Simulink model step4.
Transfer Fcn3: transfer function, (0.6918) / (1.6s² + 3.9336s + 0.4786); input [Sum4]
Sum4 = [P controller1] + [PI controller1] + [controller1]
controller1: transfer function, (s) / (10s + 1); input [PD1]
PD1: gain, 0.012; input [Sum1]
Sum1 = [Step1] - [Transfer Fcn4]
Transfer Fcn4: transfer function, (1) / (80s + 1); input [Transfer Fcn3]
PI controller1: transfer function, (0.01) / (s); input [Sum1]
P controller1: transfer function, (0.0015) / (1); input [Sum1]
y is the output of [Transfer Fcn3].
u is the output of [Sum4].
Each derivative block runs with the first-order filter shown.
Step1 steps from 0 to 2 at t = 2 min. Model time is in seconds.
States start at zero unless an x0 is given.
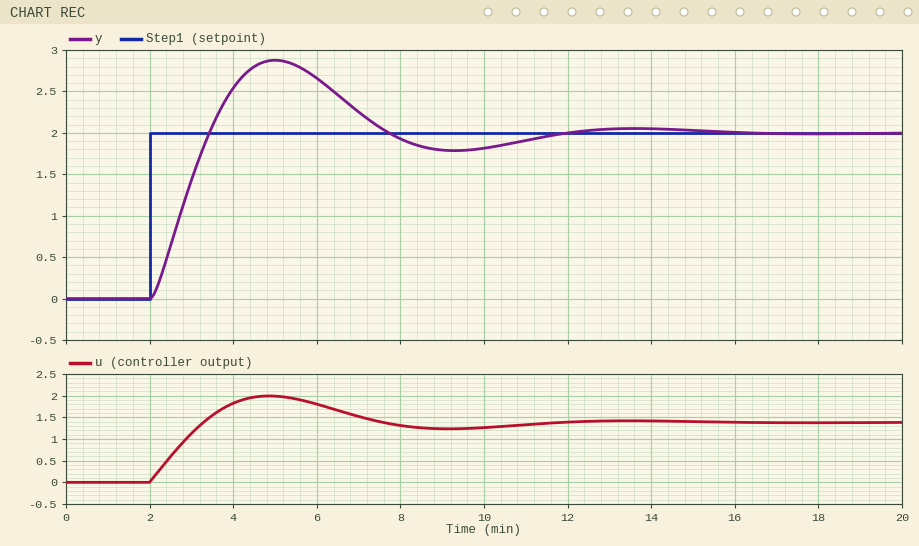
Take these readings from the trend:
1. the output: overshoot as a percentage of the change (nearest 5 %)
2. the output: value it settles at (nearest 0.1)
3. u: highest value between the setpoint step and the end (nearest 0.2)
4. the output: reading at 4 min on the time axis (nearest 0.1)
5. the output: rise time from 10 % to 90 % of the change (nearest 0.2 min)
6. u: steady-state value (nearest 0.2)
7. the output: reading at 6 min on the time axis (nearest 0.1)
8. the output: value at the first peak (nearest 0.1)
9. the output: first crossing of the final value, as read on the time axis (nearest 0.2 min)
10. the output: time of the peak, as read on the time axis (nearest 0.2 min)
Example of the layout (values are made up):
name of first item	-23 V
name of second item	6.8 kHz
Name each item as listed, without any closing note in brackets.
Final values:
the output: overshoot as a percentage of the change	45 %
the output: value it settles at	2.0
u: highest value between the setpoint step and the end	2.0
the output: reading at 4 min on the time axis	2.5
the output: rise time from 10 % to 90 % of the change	1.0 min
u: steady-state value	1.4
the output: reading at 6 min on the time axis	2.7
the output: value at the first peak	2.9
the output: first crossing of the final value, as read on the time axis	3.4 min
the output: time of the peak, as read on the time axis	5.0 min
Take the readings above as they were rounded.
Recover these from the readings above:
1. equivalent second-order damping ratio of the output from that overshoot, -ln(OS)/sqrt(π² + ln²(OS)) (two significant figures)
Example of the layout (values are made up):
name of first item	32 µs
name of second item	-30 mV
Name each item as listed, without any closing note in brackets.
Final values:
equivalent second-order damping ratio of the output from that overshoot, -ln(OS)/sqrt(π² + ln²(OS))	0.25
